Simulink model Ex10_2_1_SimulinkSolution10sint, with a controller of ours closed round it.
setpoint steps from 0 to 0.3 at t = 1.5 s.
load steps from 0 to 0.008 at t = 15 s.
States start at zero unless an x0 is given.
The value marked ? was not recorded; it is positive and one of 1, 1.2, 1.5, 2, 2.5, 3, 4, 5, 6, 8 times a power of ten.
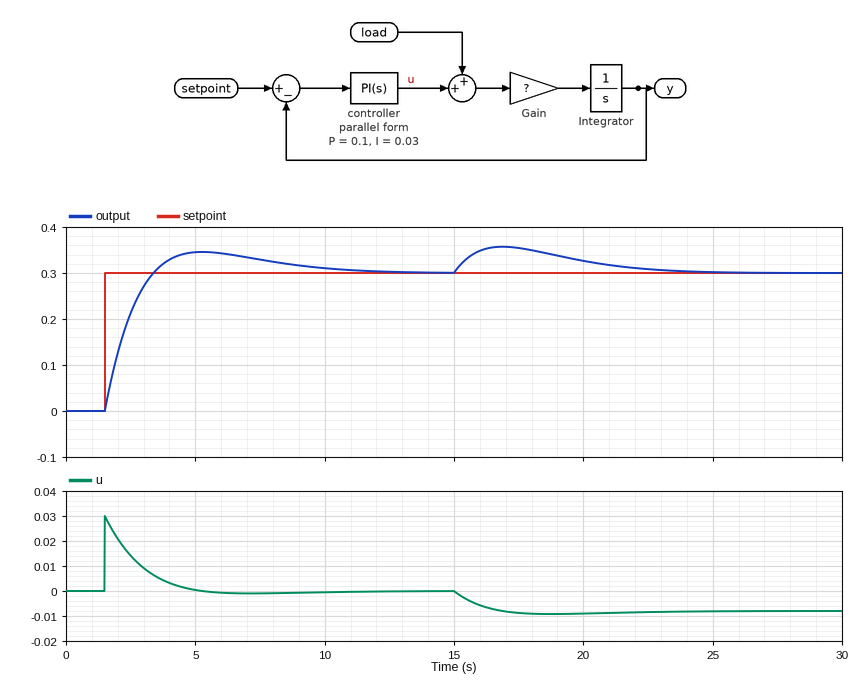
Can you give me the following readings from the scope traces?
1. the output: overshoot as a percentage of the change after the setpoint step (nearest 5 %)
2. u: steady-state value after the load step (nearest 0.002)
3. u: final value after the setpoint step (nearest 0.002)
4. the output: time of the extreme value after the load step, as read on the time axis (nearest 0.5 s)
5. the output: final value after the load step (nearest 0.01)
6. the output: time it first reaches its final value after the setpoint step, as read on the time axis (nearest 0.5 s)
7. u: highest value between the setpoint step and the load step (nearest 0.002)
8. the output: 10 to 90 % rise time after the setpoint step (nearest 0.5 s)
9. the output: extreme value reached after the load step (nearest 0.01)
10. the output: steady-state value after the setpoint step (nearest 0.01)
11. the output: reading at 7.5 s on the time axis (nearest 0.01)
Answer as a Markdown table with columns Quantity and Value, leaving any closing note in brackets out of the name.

| Quantity | Value |
|---|---|
| the output: overshoot as a percentage of the change after the setpoint step | 15 % |
| u: steady-state value after the load step | -0.008 |
| u: final value after the setpoint step | 0.000 |
| the output: time of the extreme value after the load step, as read on the time axis | 17.0 s |
| the output: final value after the load step | 0.30 |
| the output: time it first reaches its final value after the setpoint step, as read on the time axis | 3.5 s |
| u: highest value between the setpoint step and the load step | 0.030 |
| the output: 10 to 90 % rise time after the setpoint step | 1.5 s |
| the output: extreme value reached after the load step | 0.36 |
| the output: steady-state value after the setpoint step | 0.30 |
| the output: reading at 7.5 s on the time axis | 0.33 |
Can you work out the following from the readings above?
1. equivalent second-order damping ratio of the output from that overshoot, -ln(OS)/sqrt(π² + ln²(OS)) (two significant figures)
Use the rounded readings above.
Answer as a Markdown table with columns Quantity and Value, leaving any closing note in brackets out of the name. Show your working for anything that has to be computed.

| Quantity | Value |
|---|---|
| equivalent second-order damping ratio of the output from that overshoot, -ln(OS)/sqrt(π² + ln²(OS)) | ln(0.15) = -1.897; 1.897 / sqrt(9.870 + 3.599) = 0.52 |
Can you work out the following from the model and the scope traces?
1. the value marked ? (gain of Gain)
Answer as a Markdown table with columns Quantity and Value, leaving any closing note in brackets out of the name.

| Quantity | Value |
|---|---|
| the value marked ? | 10 |
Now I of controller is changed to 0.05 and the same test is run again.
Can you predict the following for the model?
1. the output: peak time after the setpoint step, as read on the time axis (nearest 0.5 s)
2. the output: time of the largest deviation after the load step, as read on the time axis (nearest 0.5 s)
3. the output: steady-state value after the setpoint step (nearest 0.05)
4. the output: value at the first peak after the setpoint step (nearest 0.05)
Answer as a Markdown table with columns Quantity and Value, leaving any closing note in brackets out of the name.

| Quantity | Value |
|---|---|
| the output: peak time after the setpoint step, as read on the time axis | 4.5 s |
| the output: time of the largest deviation after the load step, as read on the time axis | 16.5 s |
| the output: steady-state value after the setpoint step | 0.30 |
| the output: value at the first peak after the setpoint step | 0.35 |
